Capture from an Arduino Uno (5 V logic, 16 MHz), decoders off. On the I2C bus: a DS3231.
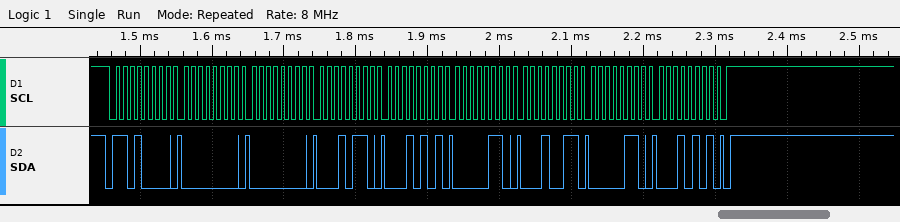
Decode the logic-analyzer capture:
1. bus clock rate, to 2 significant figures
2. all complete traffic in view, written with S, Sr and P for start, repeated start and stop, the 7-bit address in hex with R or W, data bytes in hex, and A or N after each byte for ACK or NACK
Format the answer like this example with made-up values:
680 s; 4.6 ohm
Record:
100 kHz; S 68W A 00 A 00 A 16 A 15 A 06 A 13 A 06 A 15 A P
